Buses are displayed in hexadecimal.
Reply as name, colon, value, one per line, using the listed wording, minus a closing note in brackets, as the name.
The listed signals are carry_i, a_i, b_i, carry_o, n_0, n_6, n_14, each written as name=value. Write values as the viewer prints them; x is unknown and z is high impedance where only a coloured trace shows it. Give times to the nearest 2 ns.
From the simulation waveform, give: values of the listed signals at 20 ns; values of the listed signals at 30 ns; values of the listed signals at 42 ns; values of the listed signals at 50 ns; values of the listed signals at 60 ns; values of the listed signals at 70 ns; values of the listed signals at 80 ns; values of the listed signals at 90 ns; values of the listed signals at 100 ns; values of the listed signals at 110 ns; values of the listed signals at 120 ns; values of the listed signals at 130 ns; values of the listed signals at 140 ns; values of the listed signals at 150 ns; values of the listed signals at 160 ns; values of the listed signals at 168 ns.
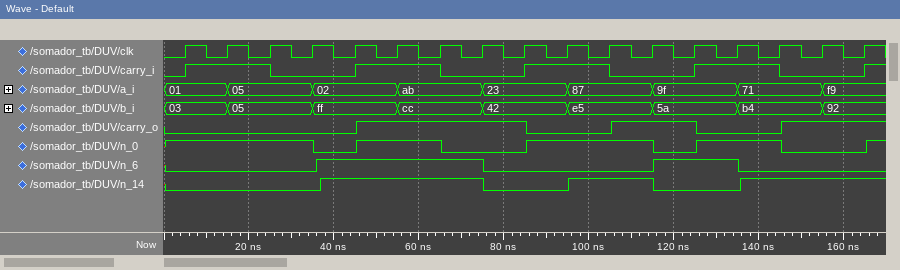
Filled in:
values of the listed signals at 20 ns: carry_i=1, a_i=05, b_i=05, carry_o=0, n_0=1, n_6=0, n_14=0
values of the listed signals at 30 ns: carry_i=0, a_i=05, b_i=05, carry_o=0, n_0=1, n_6=0, n_14=0
values of the listed signals at 42 ns: carry_i=0, a_i=02, b_i=ff, carry_o=0, n_0=0, n_6=1, n_14=1
values of the listed signals at 50 ns: carry_i=1, a_i=02, b_i=ff, carry_o=1, n_0=1, n_6=1, n_14=1
values of the listed signals at 60 ns: carry_i=1, a_i=ab, b_i=cc, carry_o=1, n_0=1, n_6=1, n_14=1
values of the listed signals at 70 ns: carry_i=0, a_i=ab, b_i=cc, carry_o=1, n_0=0, n_6=1, n_14=1
values of the listed signals at 80 ns: carry_i=0, a_i=23, b_i=42, carry_o=1, n_0=0, n_6=0, n_14=0
values of the listed signals at 90 ns: carry_i=1, a_i=23, b_i=42, carry_o=0, n_0=1, n_6=0, n_14=0
values of the listed signals at 100 ns: carry_i=1, a_i=87, b_i=e5, carry_o=0, n_0=1, n_6=0, n_14=1
values of the listed signals at 110 ns: carry_i=0, a_i=87, b_i=e5, carry_o=1, n_0=1, n_6=0, n_14=1
values of the listed signals at 120 ns: carry_i=0, a_i=9f, b_i=5a, carry_o=1, n_0=0, n_6=1, n_14=0
values of the listed signals at 130 ns: carry_i=1, a_i=9f, b_i=5a, carry_o=0, n_0=1, n_6=1, n_14=0
values of the listed signals at 140 ns: carry_i=1, a_i=71, b_i=b4, carry_o=0, n_0=1, n_6=0, n_14=1
values of the listed signals at 150 ns: carry_i=0, a_i=71, b_i=b4, carry_o=1, n_0=0, n_6=0, n_14=1
values of the listed signals at 160 ns: carry_i=0, a_i=f9, b_i=92, carry_o=1, n_0=0, n_6=0, n_14=1
values of the listed signals at 168 ns: carry_i=1, a_i=f9, b_i=92, carry_o=1, n_0=1, n_6=0, n_14=1
